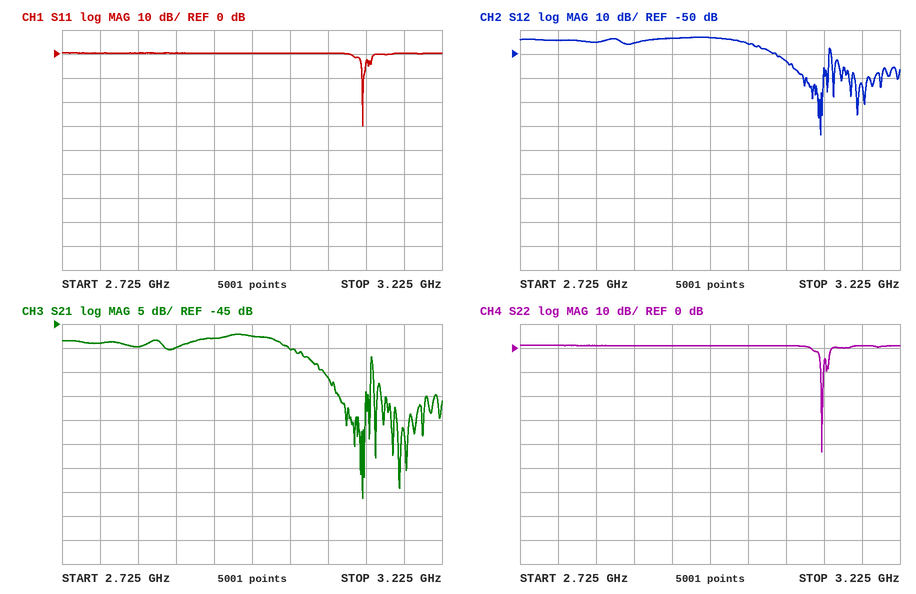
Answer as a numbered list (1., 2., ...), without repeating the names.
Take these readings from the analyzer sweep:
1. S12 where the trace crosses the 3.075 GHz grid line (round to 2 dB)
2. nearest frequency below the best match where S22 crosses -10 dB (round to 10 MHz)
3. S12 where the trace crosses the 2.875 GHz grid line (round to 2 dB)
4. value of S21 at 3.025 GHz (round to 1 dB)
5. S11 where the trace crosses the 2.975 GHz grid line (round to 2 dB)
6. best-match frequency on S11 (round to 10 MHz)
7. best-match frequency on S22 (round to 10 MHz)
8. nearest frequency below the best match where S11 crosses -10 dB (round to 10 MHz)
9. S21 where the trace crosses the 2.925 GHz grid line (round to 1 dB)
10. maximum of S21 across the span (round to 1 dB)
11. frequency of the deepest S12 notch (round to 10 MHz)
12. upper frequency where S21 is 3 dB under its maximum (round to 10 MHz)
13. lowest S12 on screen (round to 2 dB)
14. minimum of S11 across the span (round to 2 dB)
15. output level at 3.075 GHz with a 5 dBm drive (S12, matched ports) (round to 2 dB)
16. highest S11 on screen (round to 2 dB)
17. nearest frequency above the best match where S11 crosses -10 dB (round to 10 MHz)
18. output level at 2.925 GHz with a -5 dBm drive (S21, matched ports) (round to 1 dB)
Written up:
1. -52 dB
2. 3.12 GHz
3. -46 dB
4. -50 dB
5. 0 dB
6. 3.12 GHz
7. 3.12 GHz
8. 3.12 GHz
9. -48 dB
10. -47 dB
11. 3.12 GHz
12. 3.02 GHz
13. -84 dB
14. -30 dB
15. -48 dBm
16. 0 dB
17. 3.12 GHz
18. -53 dBm
